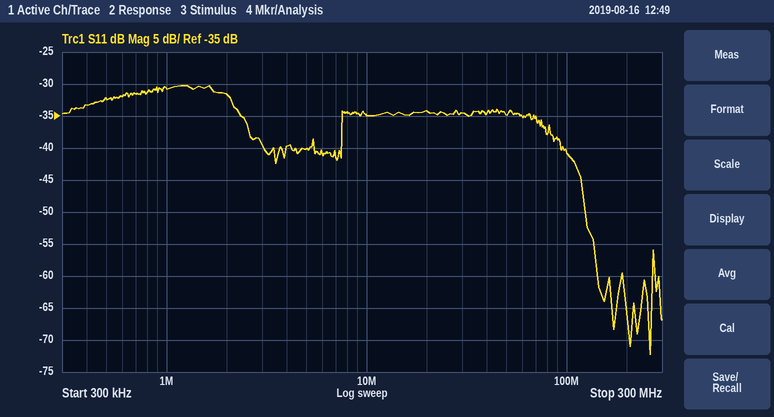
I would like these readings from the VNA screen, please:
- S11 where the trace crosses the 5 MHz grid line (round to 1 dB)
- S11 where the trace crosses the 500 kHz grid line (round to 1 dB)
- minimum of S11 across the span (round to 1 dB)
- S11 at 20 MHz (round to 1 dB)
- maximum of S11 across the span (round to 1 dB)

-40 dB
-32 dB
-72 dB
-34 dB
-30 dB
